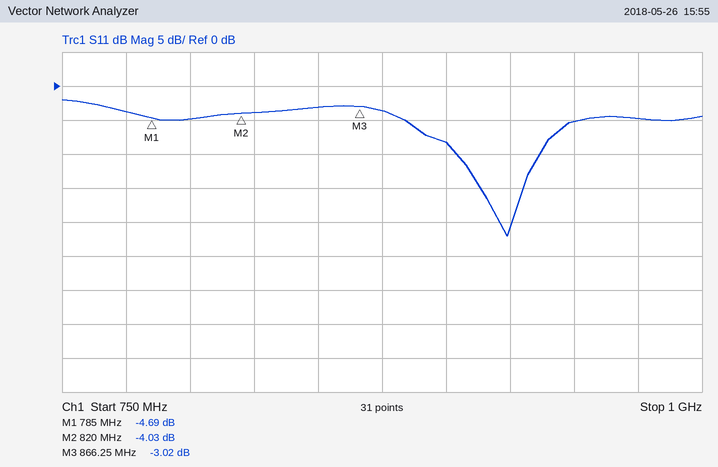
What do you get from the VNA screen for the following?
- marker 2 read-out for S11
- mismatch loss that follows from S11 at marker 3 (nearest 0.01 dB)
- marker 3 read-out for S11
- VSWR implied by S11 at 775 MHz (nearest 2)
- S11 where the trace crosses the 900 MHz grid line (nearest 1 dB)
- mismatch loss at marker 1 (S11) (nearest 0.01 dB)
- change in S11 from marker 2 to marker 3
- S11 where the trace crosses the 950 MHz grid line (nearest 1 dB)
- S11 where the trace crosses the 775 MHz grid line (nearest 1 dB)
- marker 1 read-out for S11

-4.03 dB
3.00 dB
-3.02 dB
4
-8 dB
1.80 dB
1.01 dB
-5 dB
-4 dB
-4.69 dB
